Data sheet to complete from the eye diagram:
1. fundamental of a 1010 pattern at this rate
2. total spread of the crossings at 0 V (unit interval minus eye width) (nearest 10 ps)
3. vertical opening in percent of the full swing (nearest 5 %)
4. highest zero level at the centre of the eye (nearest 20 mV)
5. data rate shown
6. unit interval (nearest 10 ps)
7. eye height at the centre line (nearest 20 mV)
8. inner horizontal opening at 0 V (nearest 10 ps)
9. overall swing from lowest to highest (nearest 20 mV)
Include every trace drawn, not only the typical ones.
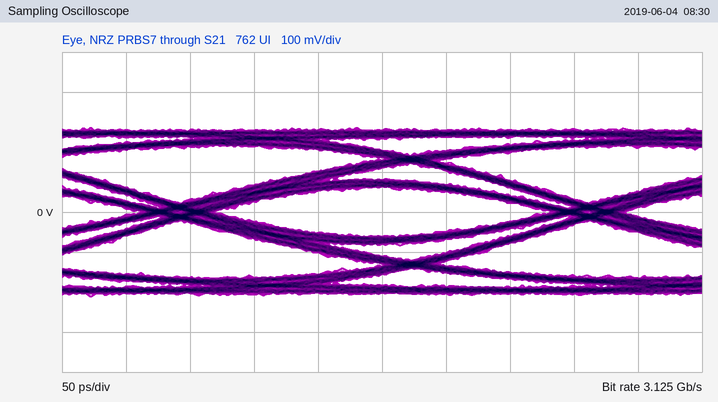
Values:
1.5625 GHz
60 ps
30 %
-60 mV
3.125 Gb/s
320 ps
120 mV
260 ps
420 mV
